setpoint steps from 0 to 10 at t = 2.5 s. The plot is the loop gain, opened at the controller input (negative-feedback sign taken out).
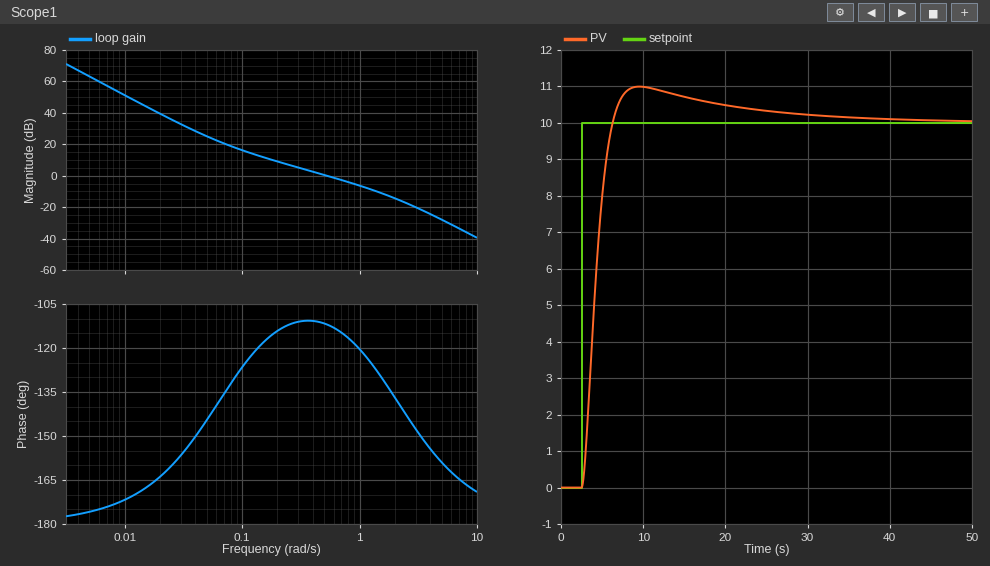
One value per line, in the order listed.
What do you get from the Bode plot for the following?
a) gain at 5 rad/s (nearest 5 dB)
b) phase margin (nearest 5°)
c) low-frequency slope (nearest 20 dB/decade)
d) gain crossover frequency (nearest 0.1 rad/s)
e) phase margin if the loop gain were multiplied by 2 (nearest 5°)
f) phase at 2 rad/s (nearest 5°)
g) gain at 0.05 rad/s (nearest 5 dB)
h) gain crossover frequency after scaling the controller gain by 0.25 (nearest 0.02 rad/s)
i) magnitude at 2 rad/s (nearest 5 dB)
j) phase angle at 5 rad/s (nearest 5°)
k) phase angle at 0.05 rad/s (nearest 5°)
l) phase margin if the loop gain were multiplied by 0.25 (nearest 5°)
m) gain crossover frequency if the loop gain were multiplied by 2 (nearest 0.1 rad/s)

-30 dB
70°
-40 dB/decade
0.5 rad/s
60°
-135°
25 dB
0.14 rad/s
-15 dB
-160°
-145°
60°
1.0 rad/s
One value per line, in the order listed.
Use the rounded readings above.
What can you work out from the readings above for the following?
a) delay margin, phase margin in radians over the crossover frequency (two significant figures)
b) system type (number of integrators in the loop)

2.4 s
2
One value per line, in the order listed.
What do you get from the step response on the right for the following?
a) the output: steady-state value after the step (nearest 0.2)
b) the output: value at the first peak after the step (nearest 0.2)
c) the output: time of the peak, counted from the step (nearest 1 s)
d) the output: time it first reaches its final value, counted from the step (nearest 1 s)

10.0
11.0
7 s
4 s
